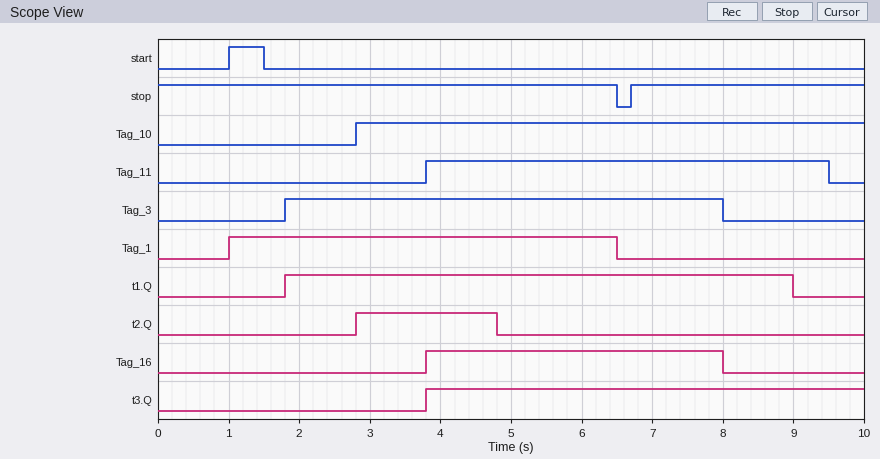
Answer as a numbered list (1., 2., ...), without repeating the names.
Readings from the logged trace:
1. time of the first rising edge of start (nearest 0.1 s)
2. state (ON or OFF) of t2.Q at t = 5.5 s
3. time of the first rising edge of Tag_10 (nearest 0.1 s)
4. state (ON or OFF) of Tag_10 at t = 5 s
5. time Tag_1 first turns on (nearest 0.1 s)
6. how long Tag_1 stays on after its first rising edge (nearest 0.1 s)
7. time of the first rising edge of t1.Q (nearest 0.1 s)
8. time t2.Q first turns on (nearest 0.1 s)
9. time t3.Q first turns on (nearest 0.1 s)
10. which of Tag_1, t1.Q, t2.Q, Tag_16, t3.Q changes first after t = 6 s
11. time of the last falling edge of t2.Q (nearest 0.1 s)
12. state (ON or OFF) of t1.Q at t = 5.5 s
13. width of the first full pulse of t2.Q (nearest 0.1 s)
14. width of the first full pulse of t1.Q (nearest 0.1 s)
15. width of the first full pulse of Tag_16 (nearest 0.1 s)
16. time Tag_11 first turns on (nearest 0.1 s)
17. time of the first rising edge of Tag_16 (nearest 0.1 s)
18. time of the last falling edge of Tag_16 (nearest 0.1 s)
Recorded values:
1. 1.0 s
2. OFF
3. 2.8 s
4. ON
5. 1.0 s
6. 5.5 s
7. 1.8 s
8. 2.8 s
9. 3.8 s
10. Tag_1
11. 4.8 s
12. ON
13. 2.0 s
14. 7.2 s
15. 4.2 s
16. 3.8 s
17. 3.8 s
18. 8.0 s
